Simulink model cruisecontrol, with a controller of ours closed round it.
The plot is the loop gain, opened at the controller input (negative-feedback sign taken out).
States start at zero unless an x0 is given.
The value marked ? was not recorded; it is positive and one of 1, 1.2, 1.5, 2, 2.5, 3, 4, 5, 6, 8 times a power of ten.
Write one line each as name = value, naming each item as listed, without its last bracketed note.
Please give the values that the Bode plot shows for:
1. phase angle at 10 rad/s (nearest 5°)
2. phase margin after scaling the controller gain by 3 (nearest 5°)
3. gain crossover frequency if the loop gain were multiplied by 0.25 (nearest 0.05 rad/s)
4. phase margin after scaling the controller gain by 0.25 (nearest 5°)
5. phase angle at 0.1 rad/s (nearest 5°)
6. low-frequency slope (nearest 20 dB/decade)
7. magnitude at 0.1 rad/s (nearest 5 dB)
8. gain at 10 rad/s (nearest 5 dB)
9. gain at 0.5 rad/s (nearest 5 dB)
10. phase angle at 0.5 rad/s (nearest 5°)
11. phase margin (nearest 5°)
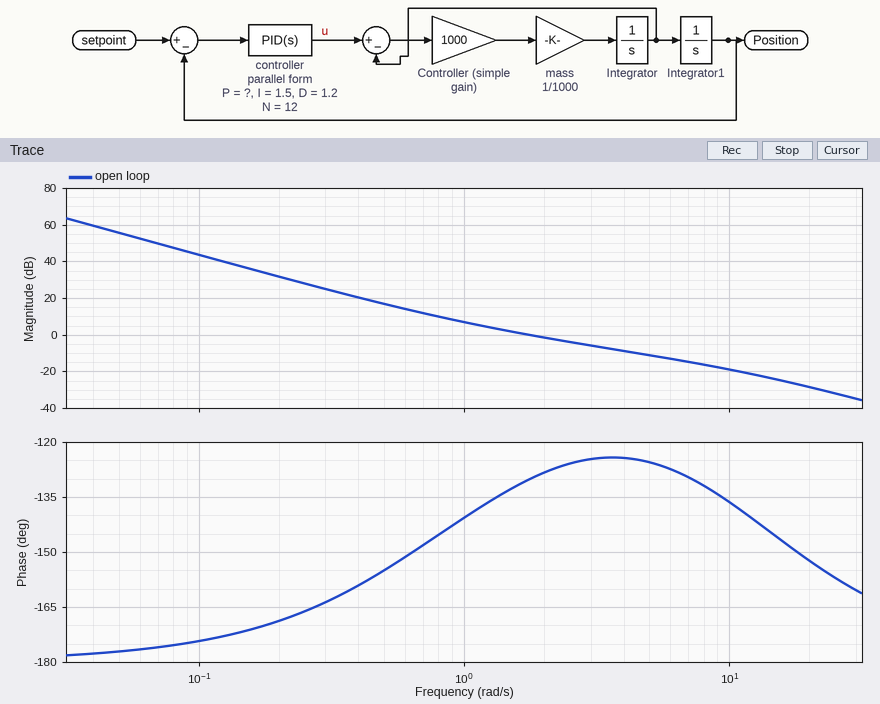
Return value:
phase angle at 10 rad/s = -135°
phase margin after scaling the controller gain by 3 = 55°
gain crossover frequency if the loop gain were multiplied by 0.25 = 0.70 rad/s
phase margin after scaling the controller gain by 0.25 = 30°
phase angle at 0.1 rad/s = -175°
low-frequency slope = -40 dB/decade
magnitude at 0.1 rad/s = 45 dB
gain at 10 rad/s = -20 dB
gain at 0.5 rad/s = 15 dB
phase angle at 0.5 rad/s = -155°
phase margin = 50°
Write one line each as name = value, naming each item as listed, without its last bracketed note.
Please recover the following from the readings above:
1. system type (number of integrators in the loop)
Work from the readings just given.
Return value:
system type = 2
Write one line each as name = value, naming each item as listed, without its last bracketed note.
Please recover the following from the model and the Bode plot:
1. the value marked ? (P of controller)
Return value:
the value marked ? = 3
